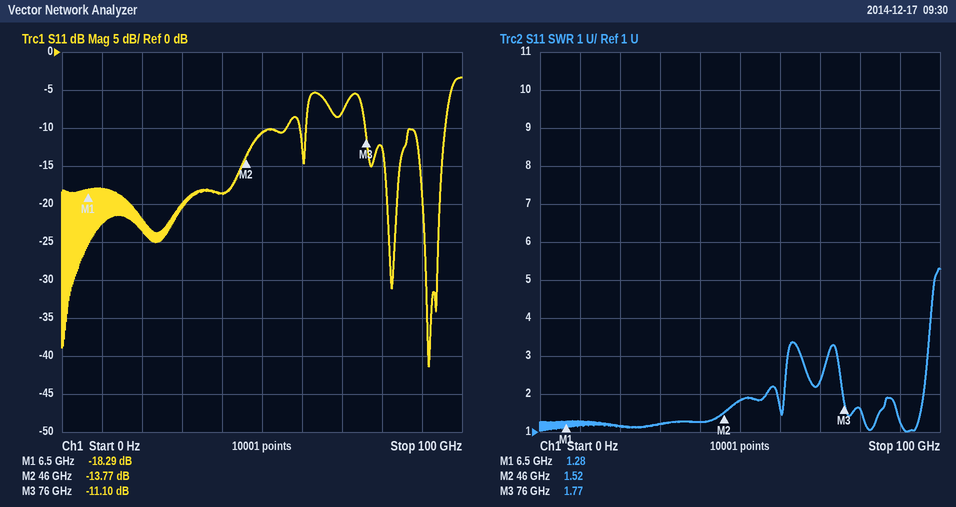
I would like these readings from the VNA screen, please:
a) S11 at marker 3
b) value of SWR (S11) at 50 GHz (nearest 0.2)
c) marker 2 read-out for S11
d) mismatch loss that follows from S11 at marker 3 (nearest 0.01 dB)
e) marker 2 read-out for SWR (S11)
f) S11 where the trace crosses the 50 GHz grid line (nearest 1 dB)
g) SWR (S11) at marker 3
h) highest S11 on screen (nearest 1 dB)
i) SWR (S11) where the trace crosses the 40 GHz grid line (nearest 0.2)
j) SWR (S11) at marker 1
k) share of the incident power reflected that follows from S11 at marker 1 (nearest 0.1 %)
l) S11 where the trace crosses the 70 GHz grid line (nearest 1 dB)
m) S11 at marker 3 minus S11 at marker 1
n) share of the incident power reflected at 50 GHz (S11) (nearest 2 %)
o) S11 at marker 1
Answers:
-11.10 dB
1.8
-13.77 dB
0.35 dB
1.52
-11 dB
1.77
-3 dB
1.2
1.28
1.5 %
-8 dB
7.19 dB
8 %
-18.29 dB
